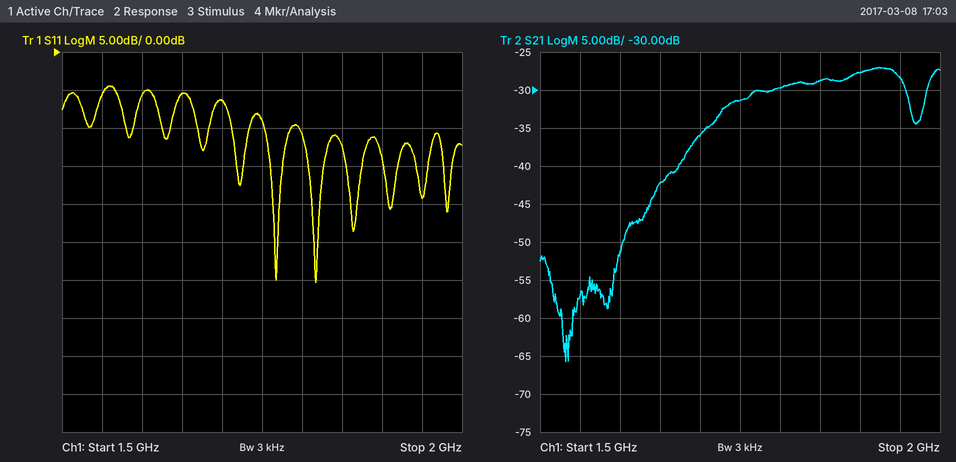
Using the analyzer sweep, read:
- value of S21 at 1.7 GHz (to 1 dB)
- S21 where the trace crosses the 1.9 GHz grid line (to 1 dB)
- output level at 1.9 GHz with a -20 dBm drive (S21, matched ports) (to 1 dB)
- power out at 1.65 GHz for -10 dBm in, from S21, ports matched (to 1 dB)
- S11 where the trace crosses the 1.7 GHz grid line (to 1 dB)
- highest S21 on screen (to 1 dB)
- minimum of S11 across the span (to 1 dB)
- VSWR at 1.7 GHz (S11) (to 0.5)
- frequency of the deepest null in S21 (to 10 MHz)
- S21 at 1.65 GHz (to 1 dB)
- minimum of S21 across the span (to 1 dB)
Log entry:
-36 dB
-28 dB
-48 dBm
-52 dBm
-6 dB
-27 dB
-30 dB
3.0
1.53 GHz
-42 dB
-66 dB
